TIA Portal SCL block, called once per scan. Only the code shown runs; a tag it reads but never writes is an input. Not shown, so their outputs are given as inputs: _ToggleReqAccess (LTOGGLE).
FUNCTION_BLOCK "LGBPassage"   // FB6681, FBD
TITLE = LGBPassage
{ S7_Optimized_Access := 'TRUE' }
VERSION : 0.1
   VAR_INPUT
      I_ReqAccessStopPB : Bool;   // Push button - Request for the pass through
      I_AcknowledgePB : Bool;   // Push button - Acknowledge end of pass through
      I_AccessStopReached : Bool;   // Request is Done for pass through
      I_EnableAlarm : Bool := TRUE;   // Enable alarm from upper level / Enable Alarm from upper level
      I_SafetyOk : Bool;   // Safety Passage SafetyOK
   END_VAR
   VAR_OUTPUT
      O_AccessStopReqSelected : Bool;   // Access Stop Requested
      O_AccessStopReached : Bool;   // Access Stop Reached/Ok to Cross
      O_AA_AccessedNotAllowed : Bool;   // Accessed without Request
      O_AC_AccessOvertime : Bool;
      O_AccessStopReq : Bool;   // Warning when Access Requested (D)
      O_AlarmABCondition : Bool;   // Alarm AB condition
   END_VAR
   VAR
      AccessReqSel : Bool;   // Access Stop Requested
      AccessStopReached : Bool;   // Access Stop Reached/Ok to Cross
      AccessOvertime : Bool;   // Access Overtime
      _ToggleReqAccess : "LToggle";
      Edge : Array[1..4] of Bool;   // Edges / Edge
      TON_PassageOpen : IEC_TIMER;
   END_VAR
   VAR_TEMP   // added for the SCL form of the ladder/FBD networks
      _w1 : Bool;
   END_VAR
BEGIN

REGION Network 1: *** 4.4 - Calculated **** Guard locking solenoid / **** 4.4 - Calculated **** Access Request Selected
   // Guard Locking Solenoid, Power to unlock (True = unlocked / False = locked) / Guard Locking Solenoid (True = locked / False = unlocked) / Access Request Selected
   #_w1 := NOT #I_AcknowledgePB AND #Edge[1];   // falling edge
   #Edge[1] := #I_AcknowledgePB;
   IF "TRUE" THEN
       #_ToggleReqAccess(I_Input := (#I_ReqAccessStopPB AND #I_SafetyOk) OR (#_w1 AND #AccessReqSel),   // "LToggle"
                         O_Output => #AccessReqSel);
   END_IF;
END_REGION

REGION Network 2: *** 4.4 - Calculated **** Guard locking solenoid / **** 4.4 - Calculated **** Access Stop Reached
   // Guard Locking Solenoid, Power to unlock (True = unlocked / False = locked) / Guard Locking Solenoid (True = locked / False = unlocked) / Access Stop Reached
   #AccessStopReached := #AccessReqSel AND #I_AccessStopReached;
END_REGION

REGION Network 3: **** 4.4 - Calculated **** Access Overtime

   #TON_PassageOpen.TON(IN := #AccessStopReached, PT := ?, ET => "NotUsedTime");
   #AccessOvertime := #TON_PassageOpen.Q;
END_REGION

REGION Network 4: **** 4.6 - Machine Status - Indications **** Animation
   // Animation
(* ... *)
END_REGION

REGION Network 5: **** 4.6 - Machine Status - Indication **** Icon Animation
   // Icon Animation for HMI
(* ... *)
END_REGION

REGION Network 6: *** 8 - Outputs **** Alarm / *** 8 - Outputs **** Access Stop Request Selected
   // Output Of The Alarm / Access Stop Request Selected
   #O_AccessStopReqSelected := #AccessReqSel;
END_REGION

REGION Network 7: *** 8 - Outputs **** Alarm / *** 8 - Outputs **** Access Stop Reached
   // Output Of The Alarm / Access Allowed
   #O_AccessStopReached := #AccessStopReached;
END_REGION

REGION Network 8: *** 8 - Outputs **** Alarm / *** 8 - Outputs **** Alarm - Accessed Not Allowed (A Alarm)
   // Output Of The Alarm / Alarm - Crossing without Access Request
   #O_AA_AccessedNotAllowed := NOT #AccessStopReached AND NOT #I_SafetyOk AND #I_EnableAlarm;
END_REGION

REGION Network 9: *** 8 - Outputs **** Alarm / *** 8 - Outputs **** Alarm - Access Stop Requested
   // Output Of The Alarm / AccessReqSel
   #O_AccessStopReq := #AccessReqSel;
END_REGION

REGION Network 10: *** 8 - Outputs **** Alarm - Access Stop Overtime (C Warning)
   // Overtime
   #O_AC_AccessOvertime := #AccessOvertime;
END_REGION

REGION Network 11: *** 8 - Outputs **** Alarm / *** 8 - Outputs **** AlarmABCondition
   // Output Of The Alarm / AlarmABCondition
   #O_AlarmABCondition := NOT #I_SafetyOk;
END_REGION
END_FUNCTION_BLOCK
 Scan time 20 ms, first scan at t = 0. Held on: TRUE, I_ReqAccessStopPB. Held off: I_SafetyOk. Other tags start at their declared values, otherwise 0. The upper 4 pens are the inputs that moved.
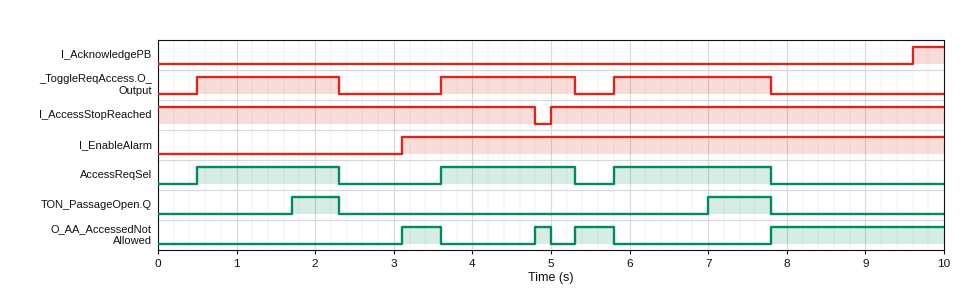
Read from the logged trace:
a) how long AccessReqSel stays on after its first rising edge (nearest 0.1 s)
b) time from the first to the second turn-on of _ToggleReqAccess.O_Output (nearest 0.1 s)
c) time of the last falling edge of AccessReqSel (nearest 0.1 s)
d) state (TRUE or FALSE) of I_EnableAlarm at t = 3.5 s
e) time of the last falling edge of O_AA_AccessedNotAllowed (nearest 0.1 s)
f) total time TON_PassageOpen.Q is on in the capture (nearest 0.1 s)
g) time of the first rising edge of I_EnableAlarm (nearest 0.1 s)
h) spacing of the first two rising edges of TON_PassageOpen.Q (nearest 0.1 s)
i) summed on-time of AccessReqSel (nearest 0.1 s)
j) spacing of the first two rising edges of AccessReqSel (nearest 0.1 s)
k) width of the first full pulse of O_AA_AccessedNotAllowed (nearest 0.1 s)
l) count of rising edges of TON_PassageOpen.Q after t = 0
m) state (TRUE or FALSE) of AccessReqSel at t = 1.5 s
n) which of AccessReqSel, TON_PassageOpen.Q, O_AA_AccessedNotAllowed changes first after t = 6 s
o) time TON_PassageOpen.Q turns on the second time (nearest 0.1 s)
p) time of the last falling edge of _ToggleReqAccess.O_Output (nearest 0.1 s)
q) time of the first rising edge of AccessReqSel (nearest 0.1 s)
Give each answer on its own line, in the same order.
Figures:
1.8 s
3.1 s
7.8 s
TRUE
5.8 s
1.4 s
3.1 s
5.3 s
5.5 s
3.1 s
0.5 s
2
TRUE
TON_PassageOpen.Q
7.0 s
7.8 s
0.5 s
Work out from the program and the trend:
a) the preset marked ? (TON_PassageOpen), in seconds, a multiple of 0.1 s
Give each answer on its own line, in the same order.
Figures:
1.2 s
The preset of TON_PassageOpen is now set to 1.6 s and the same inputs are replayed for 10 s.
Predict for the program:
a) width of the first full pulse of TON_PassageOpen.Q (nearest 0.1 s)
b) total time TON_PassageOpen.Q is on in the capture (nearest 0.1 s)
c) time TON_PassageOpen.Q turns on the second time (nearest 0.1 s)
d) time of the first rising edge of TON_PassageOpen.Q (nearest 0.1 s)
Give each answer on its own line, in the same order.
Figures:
0.2 s
0.6 s
7.4 s
2.1 s
